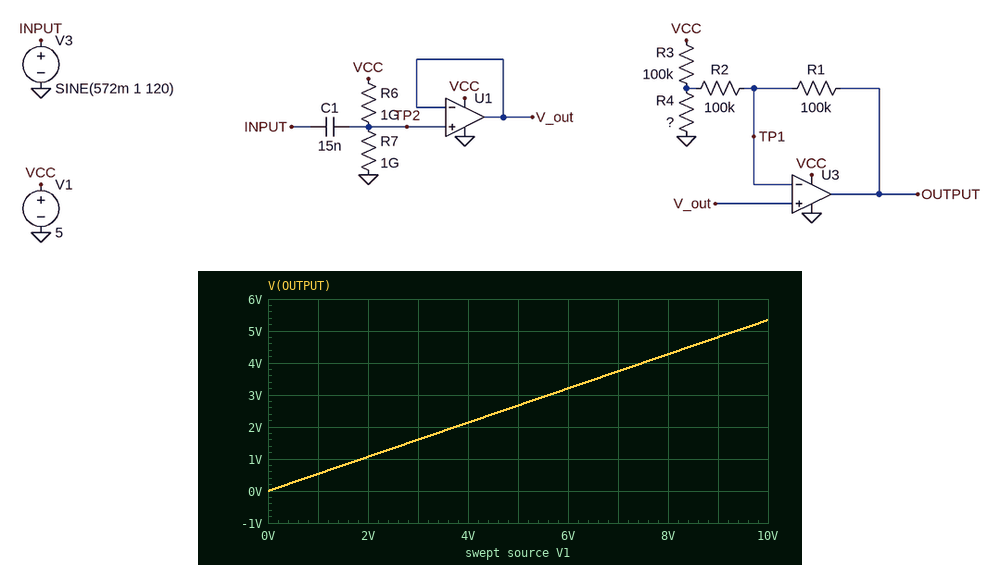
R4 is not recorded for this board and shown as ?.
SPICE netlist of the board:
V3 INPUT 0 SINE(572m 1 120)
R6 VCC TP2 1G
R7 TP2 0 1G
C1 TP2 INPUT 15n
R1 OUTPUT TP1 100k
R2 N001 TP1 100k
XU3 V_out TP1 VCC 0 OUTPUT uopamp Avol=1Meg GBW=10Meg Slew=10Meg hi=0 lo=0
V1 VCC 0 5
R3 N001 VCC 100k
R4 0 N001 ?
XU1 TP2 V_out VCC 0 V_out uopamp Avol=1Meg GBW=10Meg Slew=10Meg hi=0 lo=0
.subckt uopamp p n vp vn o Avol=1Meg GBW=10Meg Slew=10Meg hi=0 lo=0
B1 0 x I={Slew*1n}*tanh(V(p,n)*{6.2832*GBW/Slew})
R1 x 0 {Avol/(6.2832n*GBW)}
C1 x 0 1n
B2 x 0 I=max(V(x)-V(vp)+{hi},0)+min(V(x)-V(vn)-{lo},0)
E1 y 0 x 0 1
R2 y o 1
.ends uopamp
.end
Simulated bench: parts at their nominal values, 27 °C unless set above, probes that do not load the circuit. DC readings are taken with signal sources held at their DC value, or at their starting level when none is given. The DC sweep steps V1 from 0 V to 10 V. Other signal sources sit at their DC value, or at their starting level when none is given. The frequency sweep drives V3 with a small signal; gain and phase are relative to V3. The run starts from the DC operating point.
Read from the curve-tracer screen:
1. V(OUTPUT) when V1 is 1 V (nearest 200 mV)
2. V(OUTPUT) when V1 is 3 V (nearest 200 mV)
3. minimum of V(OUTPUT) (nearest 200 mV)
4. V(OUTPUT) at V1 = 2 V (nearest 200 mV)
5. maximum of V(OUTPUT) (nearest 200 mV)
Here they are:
600 mV
1.6 V
0 V
1.0 V
5.4 V
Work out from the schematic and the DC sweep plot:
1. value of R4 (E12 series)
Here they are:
82 kΩ
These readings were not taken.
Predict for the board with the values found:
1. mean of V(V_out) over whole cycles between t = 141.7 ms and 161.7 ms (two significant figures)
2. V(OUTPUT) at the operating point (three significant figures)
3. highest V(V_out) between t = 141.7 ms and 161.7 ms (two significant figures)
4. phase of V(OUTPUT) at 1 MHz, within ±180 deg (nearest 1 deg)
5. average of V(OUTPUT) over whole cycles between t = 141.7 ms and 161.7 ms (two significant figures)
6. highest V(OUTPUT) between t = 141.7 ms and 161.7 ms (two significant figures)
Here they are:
2.5 V
2.67 V
3.5 V
-15 deg
2.7 V
4.4 V
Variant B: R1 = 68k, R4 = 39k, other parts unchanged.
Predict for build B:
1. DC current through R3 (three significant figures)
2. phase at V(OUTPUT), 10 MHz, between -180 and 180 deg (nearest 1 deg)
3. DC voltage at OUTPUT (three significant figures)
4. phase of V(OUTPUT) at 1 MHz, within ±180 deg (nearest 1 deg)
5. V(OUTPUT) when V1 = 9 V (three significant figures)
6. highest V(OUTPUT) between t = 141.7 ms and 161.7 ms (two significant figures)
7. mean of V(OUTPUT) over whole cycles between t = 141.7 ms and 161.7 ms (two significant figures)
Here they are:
33.6 µA
-102 deg
3.08 V
-14 deg
5.55 V
4.6 V
3.1 V
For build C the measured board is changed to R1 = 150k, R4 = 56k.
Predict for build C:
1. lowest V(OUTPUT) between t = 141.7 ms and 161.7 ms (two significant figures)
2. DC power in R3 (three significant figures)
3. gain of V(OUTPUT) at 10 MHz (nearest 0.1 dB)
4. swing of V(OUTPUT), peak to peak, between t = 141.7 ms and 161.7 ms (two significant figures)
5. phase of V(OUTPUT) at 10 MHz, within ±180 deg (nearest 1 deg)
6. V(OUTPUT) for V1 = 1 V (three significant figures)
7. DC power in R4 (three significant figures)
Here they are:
1.2 V
91.1 µW
-3.9 dB
3.8 V
-110 deg
656 mV
70.1 µW
